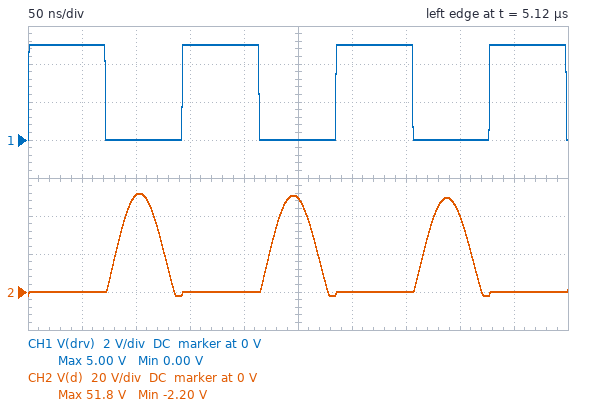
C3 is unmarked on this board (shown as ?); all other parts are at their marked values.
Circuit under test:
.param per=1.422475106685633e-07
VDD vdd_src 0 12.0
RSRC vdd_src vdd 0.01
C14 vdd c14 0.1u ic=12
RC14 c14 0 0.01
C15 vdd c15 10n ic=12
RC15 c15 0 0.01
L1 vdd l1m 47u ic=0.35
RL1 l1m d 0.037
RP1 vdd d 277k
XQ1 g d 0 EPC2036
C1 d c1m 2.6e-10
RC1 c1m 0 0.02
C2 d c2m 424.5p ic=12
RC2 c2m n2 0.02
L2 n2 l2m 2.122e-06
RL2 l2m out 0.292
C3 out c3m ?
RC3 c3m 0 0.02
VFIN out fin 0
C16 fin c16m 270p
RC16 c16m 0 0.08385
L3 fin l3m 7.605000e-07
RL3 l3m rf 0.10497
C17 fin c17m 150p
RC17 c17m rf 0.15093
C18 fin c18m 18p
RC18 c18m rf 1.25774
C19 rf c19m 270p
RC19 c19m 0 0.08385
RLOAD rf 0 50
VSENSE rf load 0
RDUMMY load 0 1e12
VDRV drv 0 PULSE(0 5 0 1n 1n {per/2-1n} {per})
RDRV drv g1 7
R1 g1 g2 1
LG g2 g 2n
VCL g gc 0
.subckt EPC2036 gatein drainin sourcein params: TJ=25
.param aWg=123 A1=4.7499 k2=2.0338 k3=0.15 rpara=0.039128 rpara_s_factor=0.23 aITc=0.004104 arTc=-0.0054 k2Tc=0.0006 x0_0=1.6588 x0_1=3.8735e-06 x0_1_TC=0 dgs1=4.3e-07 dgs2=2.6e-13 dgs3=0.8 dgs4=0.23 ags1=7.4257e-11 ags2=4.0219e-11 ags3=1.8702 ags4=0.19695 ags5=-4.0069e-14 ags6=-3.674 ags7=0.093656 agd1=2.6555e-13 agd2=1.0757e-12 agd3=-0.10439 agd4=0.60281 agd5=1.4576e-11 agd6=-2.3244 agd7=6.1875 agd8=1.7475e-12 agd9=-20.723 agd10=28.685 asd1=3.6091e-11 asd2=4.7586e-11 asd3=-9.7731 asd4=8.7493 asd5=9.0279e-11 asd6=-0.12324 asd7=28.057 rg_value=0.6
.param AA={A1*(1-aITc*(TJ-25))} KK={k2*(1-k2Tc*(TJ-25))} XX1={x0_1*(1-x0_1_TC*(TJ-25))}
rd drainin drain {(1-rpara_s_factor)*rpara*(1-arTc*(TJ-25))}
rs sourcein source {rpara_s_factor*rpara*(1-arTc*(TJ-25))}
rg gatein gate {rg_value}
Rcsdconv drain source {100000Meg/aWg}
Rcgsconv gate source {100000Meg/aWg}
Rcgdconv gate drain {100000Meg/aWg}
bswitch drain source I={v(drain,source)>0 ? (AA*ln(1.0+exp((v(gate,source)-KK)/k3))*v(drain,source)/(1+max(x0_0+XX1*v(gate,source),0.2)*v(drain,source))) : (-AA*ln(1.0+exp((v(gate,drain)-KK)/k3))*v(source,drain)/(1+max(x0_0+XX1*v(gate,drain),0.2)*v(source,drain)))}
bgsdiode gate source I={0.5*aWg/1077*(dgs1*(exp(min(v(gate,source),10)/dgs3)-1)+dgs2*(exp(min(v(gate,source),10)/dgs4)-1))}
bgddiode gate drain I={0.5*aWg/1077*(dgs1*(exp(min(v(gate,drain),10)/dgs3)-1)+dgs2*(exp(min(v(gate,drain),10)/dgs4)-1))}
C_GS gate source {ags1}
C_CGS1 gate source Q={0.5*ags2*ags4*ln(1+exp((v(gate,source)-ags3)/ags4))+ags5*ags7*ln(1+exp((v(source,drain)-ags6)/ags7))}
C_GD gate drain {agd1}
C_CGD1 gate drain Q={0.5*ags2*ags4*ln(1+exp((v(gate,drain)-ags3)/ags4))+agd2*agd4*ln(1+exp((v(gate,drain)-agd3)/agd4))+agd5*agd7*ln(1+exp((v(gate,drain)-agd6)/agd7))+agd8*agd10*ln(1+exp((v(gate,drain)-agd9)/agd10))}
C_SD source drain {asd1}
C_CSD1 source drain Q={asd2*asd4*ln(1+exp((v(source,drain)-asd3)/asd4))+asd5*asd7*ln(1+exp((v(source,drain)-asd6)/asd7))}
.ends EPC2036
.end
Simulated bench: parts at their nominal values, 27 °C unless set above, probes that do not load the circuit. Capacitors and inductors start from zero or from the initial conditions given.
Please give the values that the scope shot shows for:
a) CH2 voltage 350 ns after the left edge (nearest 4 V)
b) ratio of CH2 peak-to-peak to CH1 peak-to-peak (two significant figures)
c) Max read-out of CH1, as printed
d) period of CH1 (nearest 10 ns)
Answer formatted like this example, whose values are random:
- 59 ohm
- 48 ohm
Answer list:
- 0 V
- 11
- 5.00 V
- 140 ns
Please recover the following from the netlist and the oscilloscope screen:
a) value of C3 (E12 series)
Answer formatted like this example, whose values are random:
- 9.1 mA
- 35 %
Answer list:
- 1.8 nF
